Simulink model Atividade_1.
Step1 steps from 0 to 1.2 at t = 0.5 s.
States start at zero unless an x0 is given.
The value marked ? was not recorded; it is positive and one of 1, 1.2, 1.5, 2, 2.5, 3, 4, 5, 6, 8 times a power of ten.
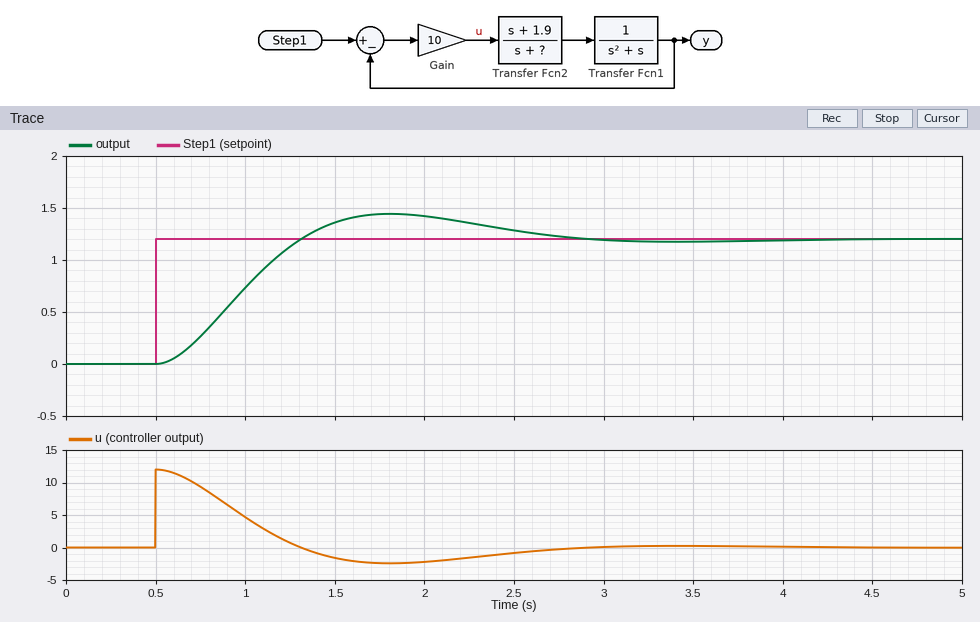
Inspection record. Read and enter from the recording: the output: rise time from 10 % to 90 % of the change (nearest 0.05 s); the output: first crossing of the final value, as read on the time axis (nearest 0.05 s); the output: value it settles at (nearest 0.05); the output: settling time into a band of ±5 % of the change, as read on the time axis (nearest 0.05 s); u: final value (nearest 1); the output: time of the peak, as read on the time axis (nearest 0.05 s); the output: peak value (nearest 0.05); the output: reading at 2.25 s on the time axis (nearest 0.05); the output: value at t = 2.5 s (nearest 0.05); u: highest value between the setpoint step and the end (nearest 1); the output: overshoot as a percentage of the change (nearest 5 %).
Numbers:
0.55 s
1.30 s
1.20
2.60 s
0
1.80 s
1.45
1.35
1.30
12
20 %
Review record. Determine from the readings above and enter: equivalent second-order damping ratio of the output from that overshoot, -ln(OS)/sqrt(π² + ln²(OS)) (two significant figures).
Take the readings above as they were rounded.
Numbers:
0.46
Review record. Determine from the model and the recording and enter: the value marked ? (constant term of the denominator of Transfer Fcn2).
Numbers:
5
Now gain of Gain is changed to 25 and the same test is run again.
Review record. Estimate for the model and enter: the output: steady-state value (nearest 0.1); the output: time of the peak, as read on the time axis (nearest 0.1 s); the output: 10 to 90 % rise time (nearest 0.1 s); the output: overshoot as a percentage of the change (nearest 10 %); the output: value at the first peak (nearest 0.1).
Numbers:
1.2
1.2 s
0.3 s
30 %
1.6
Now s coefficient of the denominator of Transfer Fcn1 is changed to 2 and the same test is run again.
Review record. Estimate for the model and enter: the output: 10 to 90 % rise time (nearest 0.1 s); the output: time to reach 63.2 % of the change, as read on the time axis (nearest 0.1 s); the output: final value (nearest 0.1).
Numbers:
0.8 s
1.1 s
1.2
